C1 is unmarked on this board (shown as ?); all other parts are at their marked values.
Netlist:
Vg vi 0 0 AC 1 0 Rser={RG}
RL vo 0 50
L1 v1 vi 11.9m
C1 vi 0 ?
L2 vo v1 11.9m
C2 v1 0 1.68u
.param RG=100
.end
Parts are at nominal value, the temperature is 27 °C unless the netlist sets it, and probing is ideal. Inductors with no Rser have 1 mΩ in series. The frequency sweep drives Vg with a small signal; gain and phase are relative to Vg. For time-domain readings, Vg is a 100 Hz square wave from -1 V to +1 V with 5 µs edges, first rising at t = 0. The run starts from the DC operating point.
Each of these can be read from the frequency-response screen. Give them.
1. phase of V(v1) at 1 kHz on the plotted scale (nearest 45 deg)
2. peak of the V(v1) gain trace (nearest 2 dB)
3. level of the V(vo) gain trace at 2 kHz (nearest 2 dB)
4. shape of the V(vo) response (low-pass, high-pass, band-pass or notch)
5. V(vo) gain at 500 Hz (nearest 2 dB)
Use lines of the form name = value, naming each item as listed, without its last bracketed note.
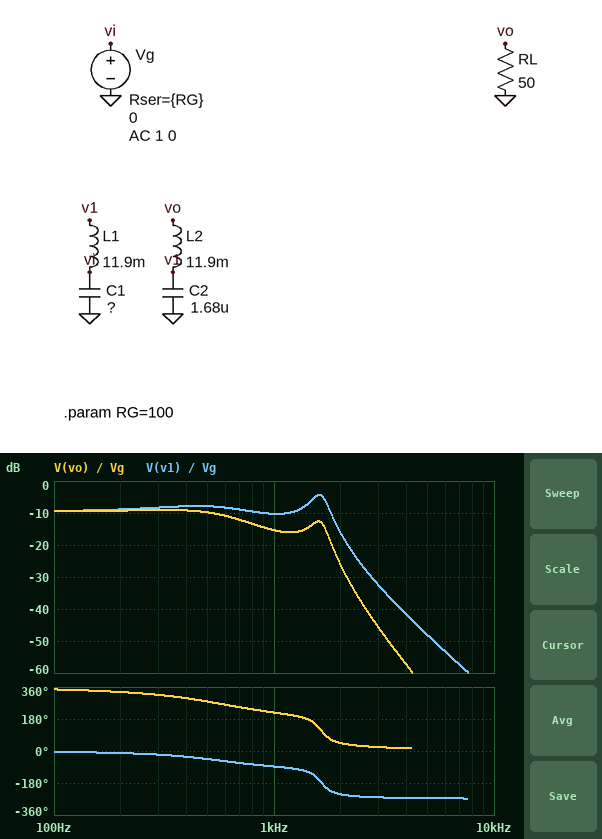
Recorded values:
phase of V(v1) at 1 kHz on the plotted scale = -90 deg
peak of the V(v1) gain trace = -4 dB
level of the V(vo) gain trace at 2 kHz = -26 dB
shape of the V(vo) response = low-pass
V(vo) gain at 500 Hz = -10 dB
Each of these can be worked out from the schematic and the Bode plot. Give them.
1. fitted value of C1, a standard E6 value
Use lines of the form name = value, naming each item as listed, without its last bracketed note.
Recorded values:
fitted value of C1, a standard E6 value = 4.7 µF
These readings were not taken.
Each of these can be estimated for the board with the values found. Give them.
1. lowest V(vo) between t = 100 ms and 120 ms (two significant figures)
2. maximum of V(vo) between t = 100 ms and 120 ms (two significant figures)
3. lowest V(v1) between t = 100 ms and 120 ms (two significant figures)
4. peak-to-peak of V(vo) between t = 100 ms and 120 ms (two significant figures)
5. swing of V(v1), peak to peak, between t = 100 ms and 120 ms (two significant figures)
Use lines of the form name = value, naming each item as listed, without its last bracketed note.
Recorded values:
lowest V(vo) between t = 100 ms and 120 ms = -420 mV
maximum of V(vo) between t = 100 ms and 120 ms = 420 mV
lowest V(v1) between t = 100 ms and 120 ms = -500 mV
peak-to-peak of V(vo) between t = 100 ms and 120 ms = 840 mV
swing of V(v1), peak to peak, between t = 100 ms and 120 ms = 1.0 V
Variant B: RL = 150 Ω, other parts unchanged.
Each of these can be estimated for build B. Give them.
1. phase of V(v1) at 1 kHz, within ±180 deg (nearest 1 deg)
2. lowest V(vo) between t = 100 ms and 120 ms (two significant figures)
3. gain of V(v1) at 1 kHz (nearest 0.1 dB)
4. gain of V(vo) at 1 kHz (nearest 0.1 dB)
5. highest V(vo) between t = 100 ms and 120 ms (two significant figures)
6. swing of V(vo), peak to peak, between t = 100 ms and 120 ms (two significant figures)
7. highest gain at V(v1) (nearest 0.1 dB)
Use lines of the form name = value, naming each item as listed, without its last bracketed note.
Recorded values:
phase of V(v1) at 1 kHz, within ±180 deg = -96 deg
lowest V(vo) between t = 100 ms and 120 ms = -610 mV
gain of V(v1) at 1 kHz = -7.6 dB
gain of V(vo) at 1 kHz = -8.6 dB
highest V(vo) between t = 100 ms and 120 ms = 610 mV
swing of V(vo), peak to peak, between t = 100 ms and 120 ms = 1.2 V
highest gain at V(v1) = -4.4 dB
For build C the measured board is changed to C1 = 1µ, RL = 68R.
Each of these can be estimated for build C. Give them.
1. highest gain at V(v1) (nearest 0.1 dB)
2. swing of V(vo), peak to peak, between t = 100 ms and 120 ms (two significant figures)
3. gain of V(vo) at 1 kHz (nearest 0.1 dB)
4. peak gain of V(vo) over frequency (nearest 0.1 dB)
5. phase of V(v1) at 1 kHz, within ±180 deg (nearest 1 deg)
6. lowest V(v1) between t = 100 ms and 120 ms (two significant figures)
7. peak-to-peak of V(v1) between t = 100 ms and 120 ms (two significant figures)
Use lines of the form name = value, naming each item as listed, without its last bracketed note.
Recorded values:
highest gain at V(v1) = -1.8 dB
swing of V(vo), peak to peak, between t = 100 ms and 120 ms = 1.0 V
gain of V(vo) at 1 kHz = -8.1 dB
peak gain of V(vo) over frequency = -7.7 dB
phase of V(v1) at 1 kHz, within ±180 deg = -49 deg
lowest V(v1) between t = 100 ms and 120 ms = -810 mV
peak-to-peak of V(v1) between t = 100 ms and 120 ms = 1.6 V
